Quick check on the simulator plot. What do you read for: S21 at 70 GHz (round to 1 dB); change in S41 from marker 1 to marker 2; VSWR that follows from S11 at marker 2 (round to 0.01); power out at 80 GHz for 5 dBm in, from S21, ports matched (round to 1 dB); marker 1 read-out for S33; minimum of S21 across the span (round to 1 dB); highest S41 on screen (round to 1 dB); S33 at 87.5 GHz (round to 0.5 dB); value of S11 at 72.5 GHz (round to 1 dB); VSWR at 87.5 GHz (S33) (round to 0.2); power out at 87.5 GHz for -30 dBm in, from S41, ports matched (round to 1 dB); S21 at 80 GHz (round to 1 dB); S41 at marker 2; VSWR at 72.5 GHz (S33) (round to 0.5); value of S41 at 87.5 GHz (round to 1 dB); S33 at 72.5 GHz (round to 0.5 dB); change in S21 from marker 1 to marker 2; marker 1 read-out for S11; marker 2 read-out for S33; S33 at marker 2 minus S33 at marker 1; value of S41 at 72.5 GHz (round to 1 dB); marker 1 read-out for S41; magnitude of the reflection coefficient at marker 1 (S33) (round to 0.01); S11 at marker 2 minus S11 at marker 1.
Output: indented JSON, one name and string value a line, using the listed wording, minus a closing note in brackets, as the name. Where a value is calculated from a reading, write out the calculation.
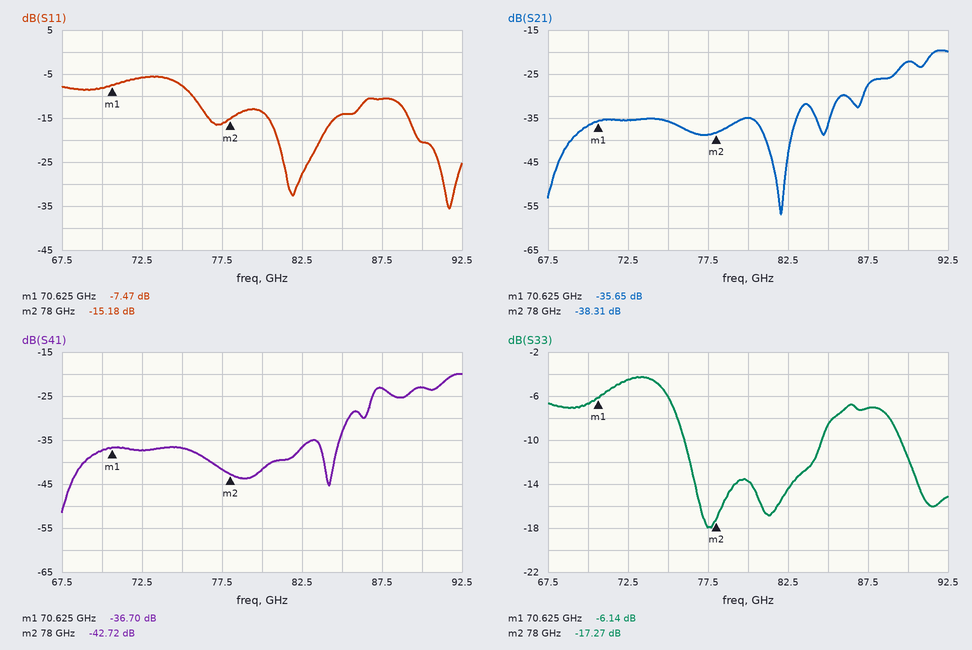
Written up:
{
  "S21 at 70 GHz": "-37 dB",
  "change in S41 from marker 1 to marker 2": "-42.72 − (-36.7) = -6.02 dB",
  "VSWR that follows from S11 at marker 2": "(1 + 0.1742)/(1 − 0.1742) ≈ 1.42",
  "power out at 80 GHz for 5 dBm in, from S21, ports matched": "5 dBm + (-35 dB) = -30 dBm",
  "marker 1 read-out for S33": "-6.14 dB",
  "minimum of S21 across the span": "-57 dB",
  "highest S41 on screen": "-20 dB",
  "S33 at 87.5 GHz": "-7.0 dB",
  "value of S11 at 72.5 GHz": "-6 dB",
  "VSWR at 87.5 GHz (S33)": "|Γ| = 10^(-7/20) = 0.4467; VSWR = (1 + 0.4467)/(1 − 0.4467) ≈ 2.6",
  "power out at 87.5 GHz for -30 dBm in, from S41, ports matched": "-30 dBm + (-23 dB) = -53 dBm",
  "S21 at 80 GHz": "-35 dB",
  "S41 at marker 2": "-42.72 dB",
  "VSWR at 72.5 GHz (S33)": "|Γ| = 10^(-4.5/20) = 0.5957; VSWR = (1 + 0.5957)/(1 − 0.5957) ≈ 4.0",
  "value of S41 at 87.5 GHz": "-23 dB",
  "S33 at 72.5 GHz": "-4.5 dB",
  "change in S21 from marker 1 to marker 2": "-38.31 − (-35.65) = -2.66 dB",
  "marker 1 read-out for S11": "-7.47 dB",
  "marker 2 read-out for S33": "-17.27 dB",
  "S33 at marker 2 minus S33 at marker 1": "-17.27 − (-6.14) = -11.13 dB",
  "value of S41 at 72.5 GHz": "-37 dB",
  "marker 1 read-out for S41": "-36.70 dB",
  "magnitude of the reflection coefficient at marker 1 (S33)": "10^(-6.14/20) ≈ 0.49",
  "S11 at marker 2 minus S11 at marker 1": "-15.18 − (-7.47) = -7.71 dB"
}
